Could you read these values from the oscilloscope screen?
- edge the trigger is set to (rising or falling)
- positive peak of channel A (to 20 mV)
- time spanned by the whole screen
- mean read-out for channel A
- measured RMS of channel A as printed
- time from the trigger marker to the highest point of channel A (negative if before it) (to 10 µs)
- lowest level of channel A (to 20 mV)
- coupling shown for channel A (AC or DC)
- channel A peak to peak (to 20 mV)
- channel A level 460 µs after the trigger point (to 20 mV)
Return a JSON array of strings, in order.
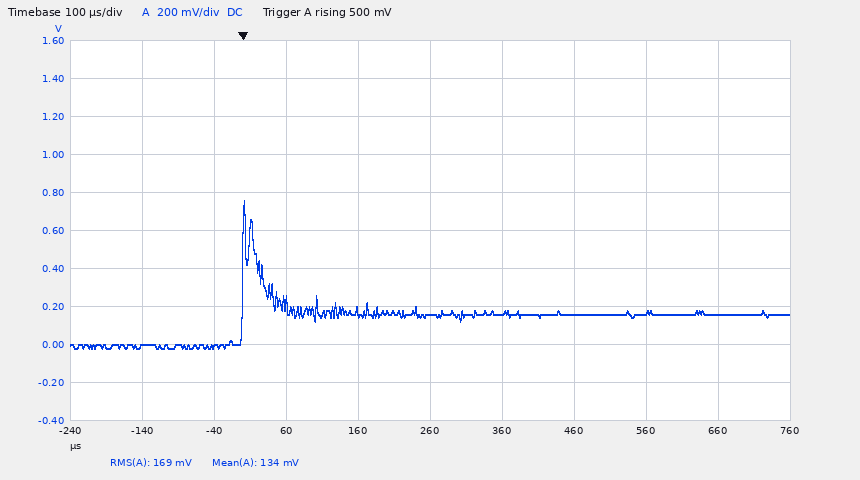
["rising", "760 mV", "1 ms", "134 mV", "169 mV", "0 µs", "-20 mV", "DC", "780 mV", "160 mV"]
